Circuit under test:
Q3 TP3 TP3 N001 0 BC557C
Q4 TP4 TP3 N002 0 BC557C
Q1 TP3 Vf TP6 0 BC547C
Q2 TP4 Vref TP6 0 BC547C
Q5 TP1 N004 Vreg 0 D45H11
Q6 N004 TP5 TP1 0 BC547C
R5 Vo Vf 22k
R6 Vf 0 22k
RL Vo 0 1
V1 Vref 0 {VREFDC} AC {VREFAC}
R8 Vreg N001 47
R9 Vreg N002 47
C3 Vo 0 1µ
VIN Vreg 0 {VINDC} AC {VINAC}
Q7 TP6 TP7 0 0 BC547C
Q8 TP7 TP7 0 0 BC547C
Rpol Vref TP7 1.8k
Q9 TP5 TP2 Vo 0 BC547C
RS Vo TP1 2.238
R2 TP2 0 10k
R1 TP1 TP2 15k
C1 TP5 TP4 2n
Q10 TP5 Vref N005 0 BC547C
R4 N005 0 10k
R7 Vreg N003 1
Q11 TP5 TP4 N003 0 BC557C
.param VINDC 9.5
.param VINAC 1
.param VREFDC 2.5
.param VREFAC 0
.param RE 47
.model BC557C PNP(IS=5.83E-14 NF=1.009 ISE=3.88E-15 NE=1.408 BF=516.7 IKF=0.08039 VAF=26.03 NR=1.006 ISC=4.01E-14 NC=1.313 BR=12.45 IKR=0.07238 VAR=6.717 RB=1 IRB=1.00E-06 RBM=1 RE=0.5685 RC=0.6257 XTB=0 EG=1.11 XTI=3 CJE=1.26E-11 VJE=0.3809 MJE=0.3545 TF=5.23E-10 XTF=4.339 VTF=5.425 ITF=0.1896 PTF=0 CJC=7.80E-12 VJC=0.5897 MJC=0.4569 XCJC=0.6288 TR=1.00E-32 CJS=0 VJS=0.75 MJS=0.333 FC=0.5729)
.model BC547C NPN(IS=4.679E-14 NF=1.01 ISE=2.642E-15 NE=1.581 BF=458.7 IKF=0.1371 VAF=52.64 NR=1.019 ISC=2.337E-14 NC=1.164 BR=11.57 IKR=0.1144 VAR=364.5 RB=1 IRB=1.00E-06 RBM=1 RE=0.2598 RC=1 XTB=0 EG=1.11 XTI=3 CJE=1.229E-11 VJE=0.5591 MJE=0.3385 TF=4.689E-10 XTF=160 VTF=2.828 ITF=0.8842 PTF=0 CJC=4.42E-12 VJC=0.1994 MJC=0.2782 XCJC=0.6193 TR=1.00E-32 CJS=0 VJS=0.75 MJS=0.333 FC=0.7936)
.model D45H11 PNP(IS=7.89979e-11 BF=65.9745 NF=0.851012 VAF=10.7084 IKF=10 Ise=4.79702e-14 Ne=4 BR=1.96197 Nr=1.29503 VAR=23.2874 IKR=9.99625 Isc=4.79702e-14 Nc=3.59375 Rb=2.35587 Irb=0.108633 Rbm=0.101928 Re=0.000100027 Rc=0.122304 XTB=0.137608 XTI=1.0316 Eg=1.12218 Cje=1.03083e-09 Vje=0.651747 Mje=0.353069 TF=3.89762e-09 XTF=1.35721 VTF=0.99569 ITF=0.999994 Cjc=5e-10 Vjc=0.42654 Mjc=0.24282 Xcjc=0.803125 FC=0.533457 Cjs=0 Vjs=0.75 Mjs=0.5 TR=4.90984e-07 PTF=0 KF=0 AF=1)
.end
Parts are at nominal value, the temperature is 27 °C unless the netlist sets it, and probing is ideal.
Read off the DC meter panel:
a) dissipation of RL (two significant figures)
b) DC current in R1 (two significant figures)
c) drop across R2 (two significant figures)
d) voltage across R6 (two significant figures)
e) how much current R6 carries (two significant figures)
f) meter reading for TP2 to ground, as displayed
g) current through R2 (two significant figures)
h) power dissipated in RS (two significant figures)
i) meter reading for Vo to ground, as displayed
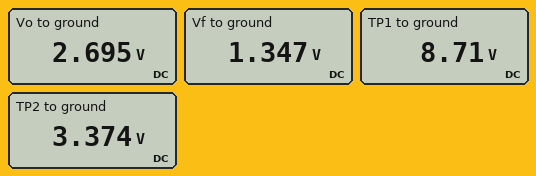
7.3 W
360 µA
3.4 V
1.3 V
61 µA
3.374 V
340 µA
16 W
2.695 V
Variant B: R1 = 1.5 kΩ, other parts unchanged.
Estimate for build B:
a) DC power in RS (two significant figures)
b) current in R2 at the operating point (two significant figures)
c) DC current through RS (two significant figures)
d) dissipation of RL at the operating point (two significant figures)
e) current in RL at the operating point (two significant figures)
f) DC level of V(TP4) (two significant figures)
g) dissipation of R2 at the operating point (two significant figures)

2.6 W
210 µA
1.1 A
1.6 W
1.3 A
8.4 V
430 µW
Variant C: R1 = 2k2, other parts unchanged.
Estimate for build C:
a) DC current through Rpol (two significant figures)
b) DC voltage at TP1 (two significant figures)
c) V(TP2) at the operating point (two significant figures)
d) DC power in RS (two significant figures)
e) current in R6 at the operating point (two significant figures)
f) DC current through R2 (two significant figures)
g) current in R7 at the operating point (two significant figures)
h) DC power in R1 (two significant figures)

1.0 mA
4.6 V
2.4 V
4.2 W
35 µA
240 µA
170 mA
2.3 mW
